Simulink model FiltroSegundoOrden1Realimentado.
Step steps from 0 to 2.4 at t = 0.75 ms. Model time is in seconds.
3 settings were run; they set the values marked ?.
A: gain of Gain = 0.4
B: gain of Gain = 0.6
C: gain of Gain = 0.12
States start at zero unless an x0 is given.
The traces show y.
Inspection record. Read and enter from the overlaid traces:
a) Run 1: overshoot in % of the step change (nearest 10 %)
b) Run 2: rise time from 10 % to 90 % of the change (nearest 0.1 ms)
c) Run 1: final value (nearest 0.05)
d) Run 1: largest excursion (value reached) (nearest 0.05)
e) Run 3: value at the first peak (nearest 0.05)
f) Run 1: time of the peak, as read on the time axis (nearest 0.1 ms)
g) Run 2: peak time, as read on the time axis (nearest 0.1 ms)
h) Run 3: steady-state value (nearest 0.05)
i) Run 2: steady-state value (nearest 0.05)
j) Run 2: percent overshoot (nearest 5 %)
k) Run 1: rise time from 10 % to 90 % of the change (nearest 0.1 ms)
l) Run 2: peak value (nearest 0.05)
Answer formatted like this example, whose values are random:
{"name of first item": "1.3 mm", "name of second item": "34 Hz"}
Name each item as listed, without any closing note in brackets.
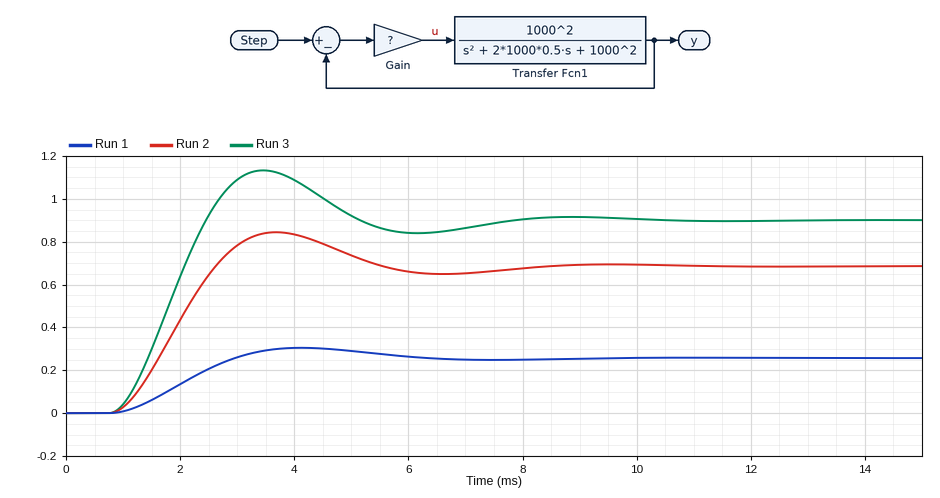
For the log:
{"Run 1: overshoot in % of the step change": "20 %", "Run 2: rise time from 10 % to 90 % of the change": "1.3 ms", "Run 1: final value": "0.25", "Run 1: largest excursion (value reached)": "0.30", "Run 3: value at the first peak": "1.15", "Run 1: time of the peak, as read on the time axis": "4.1 ms", "Run 2: peak time, as read on the time axis": "3.7 ms", "Run 3: steady-state value": "0.90", "Run 2: steady-state value": "0.70", "Run 2: percent overshoot": "25 %", "Run 1: rise time from 10 % to 90 % of the change": "1.5 ms", "Run 2: peak value": "0.85"}
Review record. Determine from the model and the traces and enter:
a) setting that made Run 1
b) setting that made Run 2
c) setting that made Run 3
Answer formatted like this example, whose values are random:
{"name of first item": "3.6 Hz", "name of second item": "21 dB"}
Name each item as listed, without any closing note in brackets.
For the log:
{"setting that made Run 1": "C", "setting that made Run 2": "A", "setting that made Run 3": "B"}
